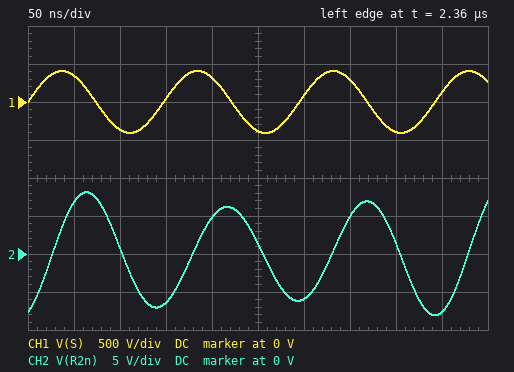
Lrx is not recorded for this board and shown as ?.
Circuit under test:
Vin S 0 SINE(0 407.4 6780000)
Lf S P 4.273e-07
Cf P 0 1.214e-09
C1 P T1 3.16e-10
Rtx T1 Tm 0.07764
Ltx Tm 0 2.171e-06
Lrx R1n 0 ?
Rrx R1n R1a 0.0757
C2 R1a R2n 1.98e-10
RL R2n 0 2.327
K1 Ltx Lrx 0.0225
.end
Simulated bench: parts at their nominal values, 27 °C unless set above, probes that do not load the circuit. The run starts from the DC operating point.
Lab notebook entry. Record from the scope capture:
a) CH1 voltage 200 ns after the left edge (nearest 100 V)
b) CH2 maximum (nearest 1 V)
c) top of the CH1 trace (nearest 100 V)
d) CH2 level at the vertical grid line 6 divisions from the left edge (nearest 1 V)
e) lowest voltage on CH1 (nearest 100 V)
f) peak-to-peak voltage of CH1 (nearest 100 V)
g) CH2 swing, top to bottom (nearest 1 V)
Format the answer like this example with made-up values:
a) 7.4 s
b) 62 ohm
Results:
a) 300 V
b) 8 V
c) 400 V
d) -6 V
e) -400 V
f) 800 V
g) 16 V
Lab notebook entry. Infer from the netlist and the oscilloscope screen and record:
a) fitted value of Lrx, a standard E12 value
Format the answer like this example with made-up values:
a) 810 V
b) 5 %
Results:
a) 3.3 µH
